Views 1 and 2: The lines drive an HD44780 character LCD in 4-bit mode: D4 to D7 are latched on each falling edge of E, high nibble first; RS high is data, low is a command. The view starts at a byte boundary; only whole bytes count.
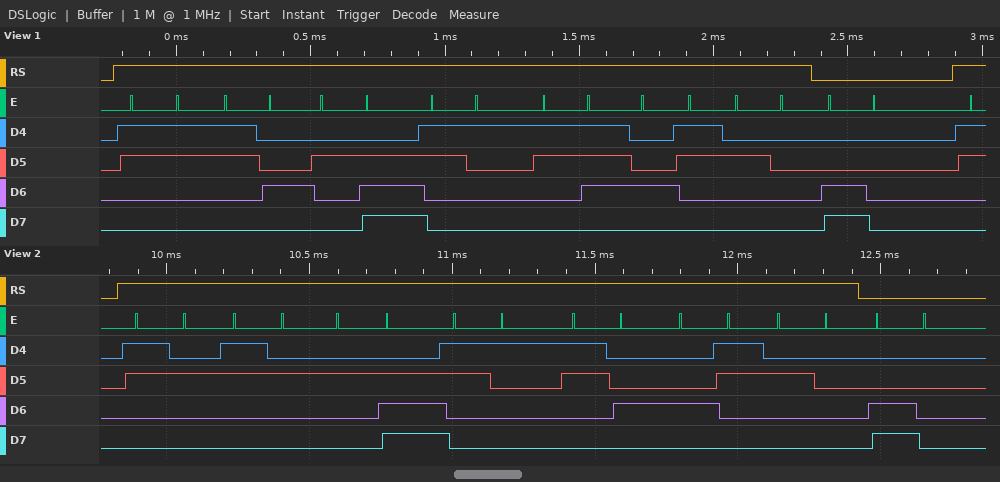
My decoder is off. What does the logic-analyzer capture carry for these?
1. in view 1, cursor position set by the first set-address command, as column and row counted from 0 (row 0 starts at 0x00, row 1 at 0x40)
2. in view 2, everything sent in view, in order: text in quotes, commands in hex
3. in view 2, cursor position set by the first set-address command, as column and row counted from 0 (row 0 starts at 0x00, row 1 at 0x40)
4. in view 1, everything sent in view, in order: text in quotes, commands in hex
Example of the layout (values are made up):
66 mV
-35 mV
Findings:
column 0, row 1
"22.14C " 0xC0
column 0, row 1
"34.17C " 0xC0
